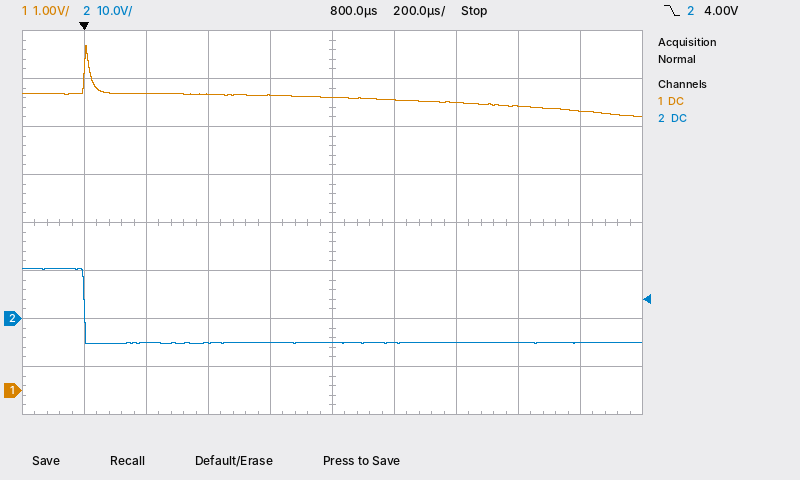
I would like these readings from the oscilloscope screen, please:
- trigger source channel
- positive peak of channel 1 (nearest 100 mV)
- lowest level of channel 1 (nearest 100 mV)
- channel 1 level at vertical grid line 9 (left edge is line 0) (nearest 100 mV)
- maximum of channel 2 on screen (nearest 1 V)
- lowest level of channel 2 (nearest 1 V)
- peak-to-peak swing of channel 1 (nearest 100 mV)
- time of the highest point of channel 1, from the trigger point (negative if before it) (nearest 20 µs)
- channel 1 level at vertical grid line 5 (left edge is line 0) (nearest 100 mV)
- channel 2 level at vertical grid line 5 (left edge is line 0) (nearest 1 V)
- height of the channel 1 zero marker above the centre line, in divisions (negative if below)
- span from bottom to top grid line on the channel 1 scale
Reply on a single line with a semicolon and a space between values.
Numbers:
channel 2; 7.2 V; 5.7 V; 5.8 V; 10 V; -5 V; 1.5 V; 0 µs; 6.1 V; -5 V; -3.5 div; 8 V
